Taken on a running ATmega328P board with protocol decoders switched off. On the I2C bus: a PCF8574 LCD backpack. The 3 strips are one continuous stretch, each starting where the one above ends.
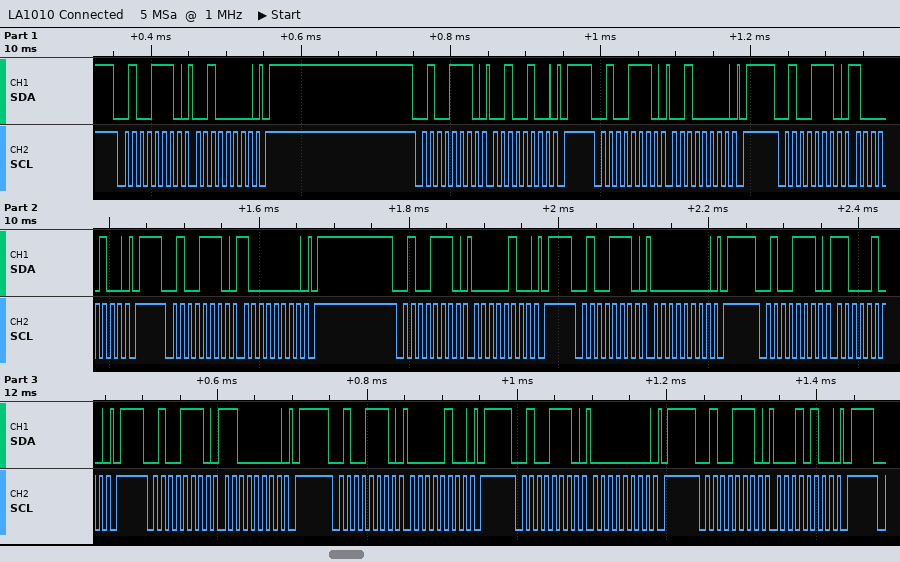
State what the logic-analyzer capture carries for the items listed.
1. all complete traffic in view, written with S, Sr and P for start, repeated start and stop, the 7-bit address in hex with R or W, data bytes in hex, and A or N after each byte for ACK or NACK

S 27W A 20 A P S 27W A 24 A P S 27W A 20 A P S 27W A 84 A P S 27W A 80 A P S 27W A 04 A P S 27W A 00 A P S 27W A C4 A P S 27W A C0 A P S 27W A 04 A P S 27W A 00 A P S 27W A 14 A P
